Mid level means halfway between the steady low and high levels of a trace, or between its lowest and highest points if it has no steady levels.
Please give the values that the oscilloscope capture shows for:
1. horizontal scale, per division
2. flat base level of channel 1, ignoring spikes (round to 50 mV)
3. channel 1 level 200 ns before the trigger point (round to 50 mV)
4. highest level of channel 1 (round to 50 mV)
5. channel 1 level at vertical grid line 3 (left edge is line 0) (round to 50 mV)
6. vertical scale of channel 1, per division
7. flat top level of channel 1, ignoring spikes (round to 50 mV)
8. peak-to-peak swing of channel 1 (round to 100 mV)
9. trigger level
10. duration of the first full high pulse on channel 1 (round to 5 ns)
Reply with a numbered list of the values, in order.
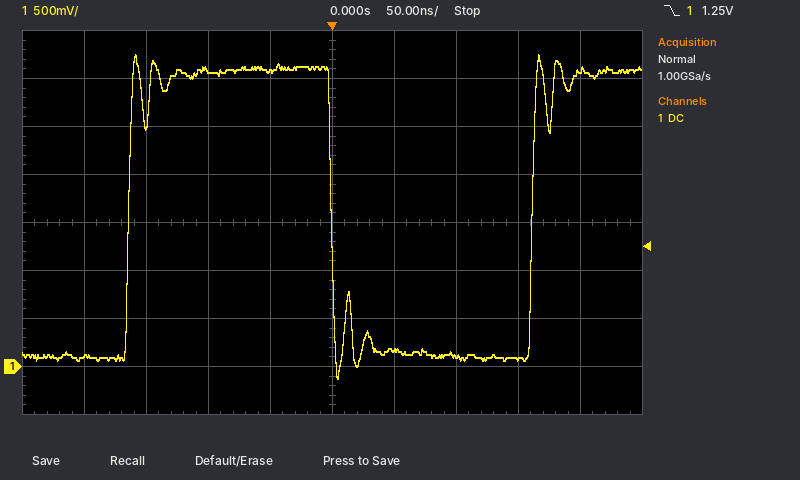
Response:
1. 50 ns
2. 100 mV
3. 100 mV
4. 3.25 V
5. 3.10 V
6. 500 mV
7. 3.10 V
8. 3.40 V
9. 1.25 V
10. 165 ns
